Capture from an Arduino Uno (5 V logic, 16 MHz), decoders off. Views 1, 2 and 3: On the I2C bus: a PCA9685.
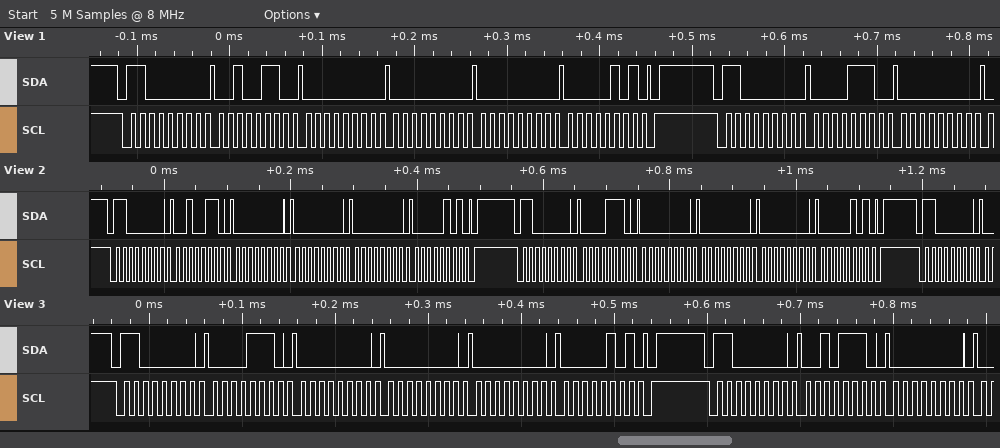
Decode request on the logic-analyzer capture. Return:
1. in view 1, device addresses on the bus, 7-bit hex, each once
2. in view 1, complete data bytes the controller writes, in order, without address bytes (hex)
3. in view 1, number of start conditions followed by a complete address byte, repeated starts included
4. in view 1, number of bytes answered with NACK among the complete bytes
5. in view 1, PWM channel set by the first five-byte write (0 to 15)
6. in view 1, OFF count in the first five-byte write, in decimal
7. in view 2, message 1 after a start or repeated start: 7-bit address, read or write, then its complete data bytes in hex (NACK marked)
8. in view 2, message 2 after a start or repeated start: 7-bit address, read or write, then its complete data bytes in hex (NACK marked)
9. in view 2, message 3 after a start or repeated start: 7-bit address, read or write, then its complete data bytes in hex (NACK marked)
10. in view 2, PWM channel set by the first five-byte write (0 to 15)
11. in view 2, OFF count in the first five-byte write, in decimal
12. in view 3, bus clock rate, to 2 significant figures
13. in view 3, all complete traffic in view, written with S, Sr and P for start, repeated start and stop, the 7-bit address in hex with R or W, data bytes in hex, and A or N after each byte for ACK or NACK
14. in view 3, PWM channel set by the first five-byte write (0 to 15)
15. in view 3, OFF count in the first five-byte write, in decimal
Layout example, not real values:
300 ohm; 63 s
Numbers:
0x60; 26 00 00 00 05 0E 00; 2; 0; 8; 1280; 0x60 write: 26 00 00 00 05; 0x60 write: 0E 00 00 00 05; 0x60 write; 8; 1280; 100 kHz; S 60W A 0E A 00 A 00 A 00 A 05 A P S 60W A 2E A 00 A; 2; 1280
